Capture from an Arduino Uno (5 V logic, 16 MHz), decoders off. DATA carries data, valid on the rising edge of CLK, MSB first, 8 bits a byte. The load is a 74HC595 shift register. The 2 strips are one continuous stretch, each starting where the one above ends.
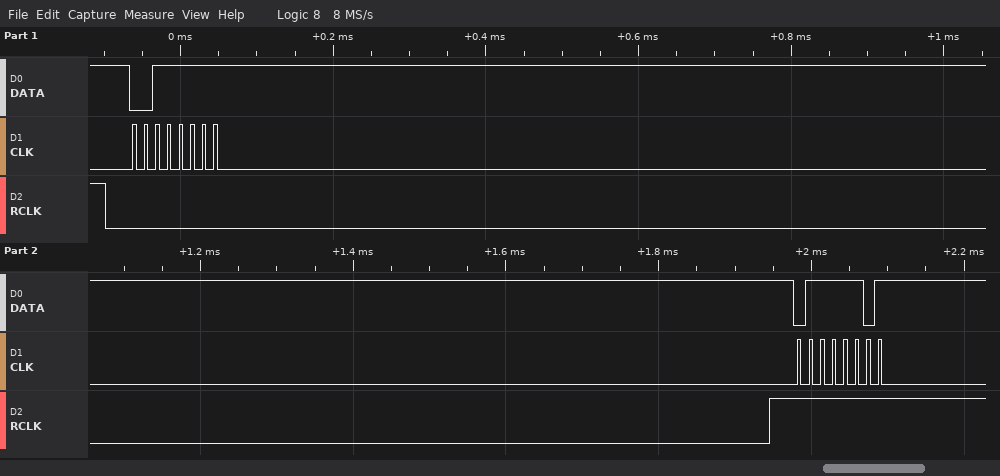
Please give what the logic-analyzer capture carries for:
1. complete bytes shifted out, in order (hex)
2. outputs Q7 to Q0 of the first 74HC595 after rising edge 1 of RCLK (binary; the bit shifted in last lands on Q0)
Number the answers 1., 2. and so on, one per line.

1. 0x3F 0x7D
2. 00111111
